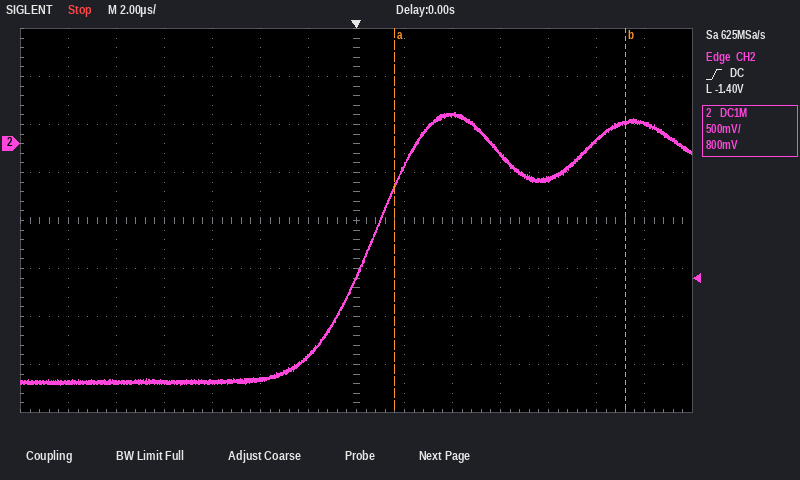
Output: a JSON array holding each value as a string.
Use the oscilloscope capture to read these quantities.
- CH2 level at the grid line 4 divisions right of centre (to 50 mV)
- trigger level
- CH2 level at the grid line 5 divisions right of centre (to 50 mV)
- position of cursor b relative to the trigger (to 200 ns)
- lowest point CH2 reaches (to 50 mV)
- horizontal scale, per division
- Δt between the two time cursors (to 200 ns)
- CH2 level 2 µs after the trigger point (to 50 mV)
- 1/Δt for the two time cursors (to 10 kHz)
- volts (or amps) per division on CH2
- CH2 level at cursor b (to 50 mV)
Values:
["-350 mV", "-1.40 V", "50 mV", "+11.2 µs", "-2.50 V", "2 µs", "9.6 µs", "-250 mV", "100 kHz", "500 mV", "200 mV"]
